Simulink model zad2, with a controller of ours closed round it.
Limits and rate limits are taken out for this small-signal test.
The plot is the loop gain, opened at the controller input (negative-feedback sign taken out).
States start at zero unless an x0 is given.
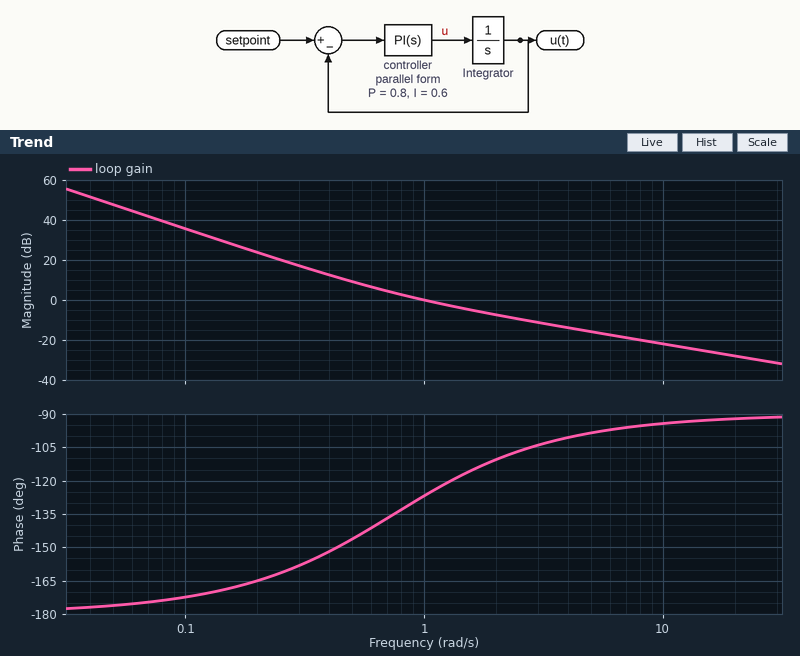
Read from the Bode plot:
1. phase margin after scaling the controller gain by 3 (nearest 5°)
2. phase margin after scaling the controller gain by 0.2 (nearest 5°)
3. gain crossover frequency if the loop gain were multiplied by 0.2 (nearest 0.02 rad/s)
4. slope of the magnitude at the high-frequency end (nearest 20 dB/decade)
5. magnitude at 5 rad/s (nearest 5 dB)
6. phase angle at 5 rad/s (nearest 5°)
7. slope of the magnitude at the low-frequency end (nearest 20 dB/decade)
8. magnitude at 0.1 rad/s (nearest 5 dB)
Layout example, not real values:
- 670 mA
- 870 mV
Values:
- 75°
- 25°
- 0.36 rad/s
- -20 dB/decade
- -15 dB
- -100°
- -40 dB/decade
- 35 dB
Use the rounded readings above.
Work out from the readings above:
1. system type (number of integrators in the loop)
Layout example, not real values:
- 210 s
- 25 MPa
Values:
- 2
